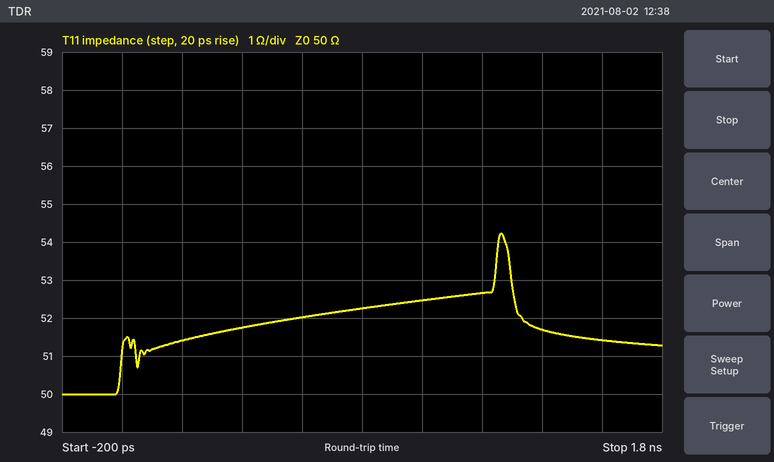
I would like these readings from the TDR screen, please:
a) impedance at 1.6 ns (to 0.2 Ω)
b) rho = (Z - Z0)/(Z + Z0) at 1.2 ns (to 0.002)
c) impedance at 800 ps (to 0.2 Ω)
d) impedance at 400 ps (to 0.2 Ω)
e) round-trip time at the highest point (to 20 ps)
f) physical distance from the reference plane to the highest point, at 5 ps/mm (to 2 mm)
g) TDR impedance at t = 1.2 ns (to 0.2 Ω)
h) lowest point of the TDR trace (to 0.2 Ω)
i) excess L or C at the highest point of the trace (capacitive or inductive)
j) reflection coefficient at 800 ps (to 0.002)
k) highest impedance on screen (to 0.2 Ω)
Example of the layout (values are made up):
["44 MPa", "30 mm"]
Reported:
["51.4 Ω", "+0.026", "52.2 Ω", "51.8 Ω", "1.26 ns", "126 mm", "52.6 Ω", "50.0 Ω", "inductive", "+0.022", "54.2 Ω"]
